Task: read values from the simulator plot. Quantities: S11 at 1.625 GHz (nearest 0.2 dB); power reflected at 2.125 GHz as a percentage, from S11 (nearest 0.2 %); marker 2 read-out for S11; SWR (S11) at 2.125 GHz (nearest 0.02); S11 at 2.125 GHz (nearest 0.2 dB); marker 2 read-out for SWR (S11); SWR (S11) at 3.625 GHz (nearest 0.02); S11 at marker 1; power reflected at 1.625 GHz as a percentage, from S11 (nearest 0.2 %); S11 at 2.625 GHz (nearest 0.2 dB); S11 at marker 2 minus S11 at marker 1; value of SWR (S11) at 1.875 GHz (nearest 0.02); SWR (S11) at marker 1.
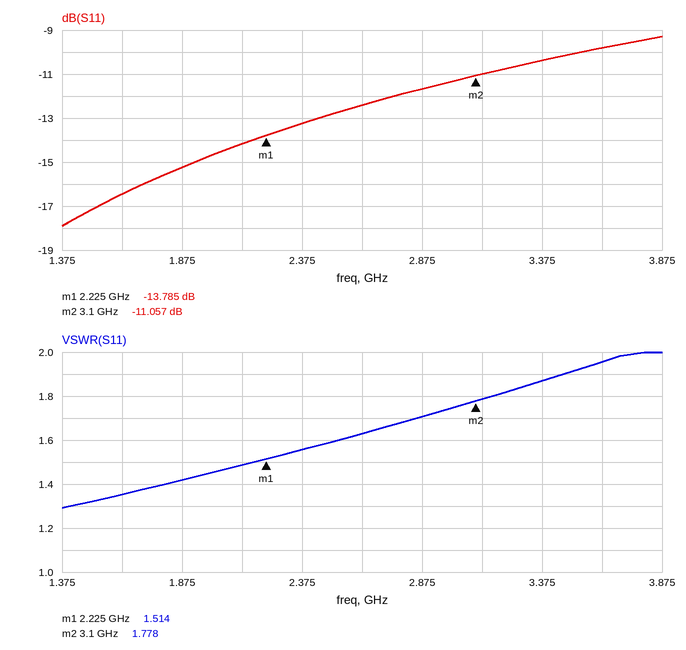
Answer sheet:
-16.4 dB
3.8 %
-11.057 dB
1.48
-14.2 dB
1.778
1.96
-13.785 dB
2.2 %
-12.4 dB
2.728 dB
1.42
1.514
